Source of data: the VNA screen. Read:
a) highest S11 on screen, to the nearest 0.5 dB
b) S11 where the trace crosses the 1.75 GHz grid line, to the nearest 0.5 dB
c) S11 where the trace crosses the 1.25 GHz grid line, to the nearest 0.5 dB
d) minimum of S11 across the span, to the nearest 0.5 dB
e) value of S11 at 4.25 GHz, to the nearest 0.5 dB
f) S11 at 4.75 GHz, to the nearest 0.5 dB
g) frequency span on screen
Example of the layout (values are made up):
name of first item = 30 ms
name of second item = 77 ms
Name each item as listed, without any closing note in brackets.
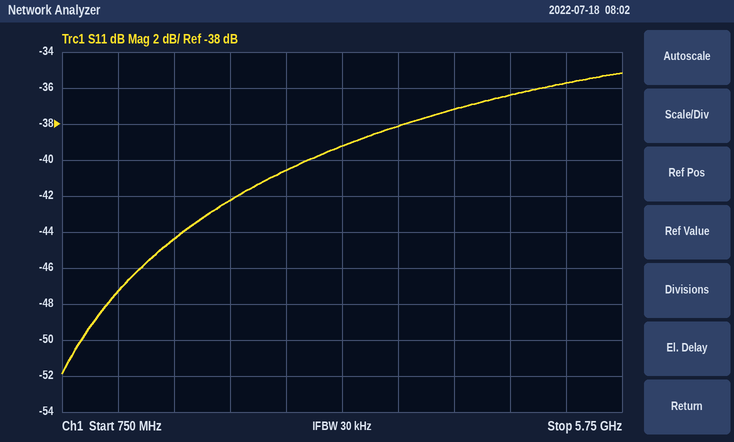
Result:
highest S11 on screen, to the nearest 0.5 dB = -35.0 dB
S11 where the trace crosses the 1.75 GHz grid line, to the nearest 0.5 dB = -44.5 dB
S11 where the trace crosses the 1.25 GHz grid line, to the nearest 0.5 dB = -47.5 dB
minimum of S11 across the span, to the nearest 0.5 dB = -52.0 dB
value of S11 at 4.25 GHz, to the nearest 0.5 dB = -37.0 dB
S11 at 4.75 GHz, to the nearest 0.5 dB = -36.5 dB
frequency span on screen = 5 GHz
